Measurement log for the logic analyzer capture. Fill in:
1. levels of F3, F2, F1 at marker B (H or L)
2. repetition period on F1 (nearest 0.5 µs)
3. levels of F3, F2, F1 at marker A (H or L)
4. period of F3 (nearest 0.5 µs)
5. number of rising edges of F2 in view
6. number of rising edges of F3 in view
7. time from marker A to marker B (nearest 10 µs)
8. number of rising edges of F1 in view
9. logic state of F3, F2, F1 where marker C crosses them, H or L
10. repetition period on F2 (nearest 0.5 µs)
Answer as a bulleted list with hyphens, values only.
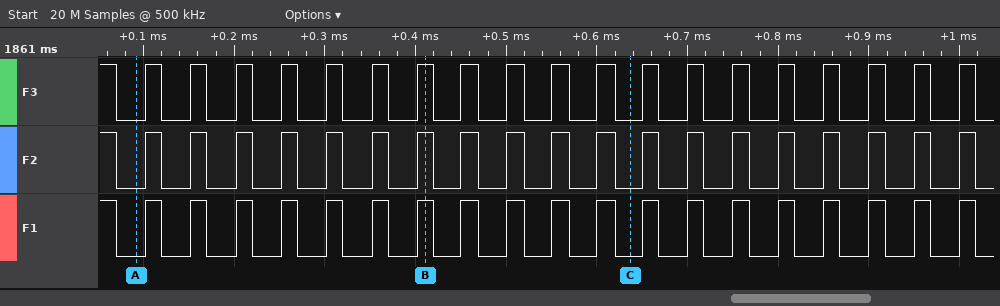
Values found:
- F3=H, F2=H, F1=H
- 50 µs
- F3=L, F2=L, F1=L
- 50 µs
- 19
- 19
- 320 µs
- 19
- F3=L, F2=L, F1=L
- 50 µs
